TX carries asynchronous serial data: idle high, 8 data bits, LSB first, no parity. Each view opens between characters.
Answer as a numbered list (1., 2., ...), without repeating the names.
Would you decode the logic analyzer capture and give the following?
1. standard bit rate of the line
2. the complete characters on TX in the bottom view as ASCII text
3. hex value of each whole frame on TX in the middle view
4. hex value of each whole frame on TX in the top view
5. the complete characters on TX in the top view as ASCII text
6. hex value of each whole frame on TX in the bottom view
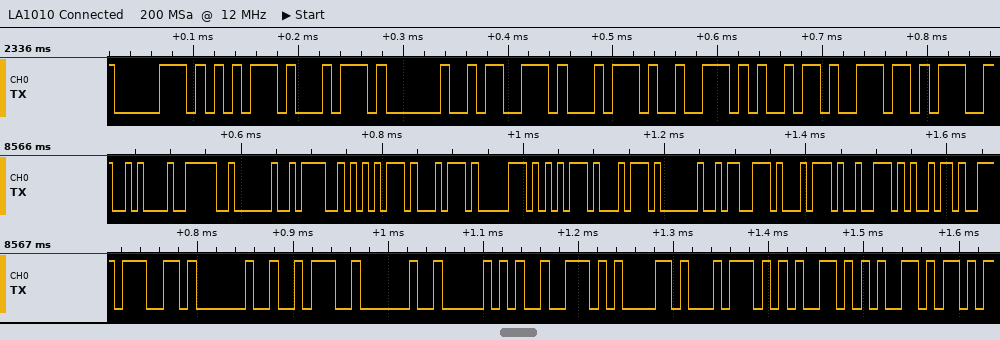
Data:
1. 115200 baud
2. "g : Pratee"
3. 0A, 3E, 20, 4F, 75, 74, 70, 75, 74, 20, 73, 74, 72, 69
4. 70, 75, 74, 20, 73, 74, 72, 69, 6E
5. "put strin"
6. 67, 20, 3A, 20, 50, 72, 61, 74, 65, 65
